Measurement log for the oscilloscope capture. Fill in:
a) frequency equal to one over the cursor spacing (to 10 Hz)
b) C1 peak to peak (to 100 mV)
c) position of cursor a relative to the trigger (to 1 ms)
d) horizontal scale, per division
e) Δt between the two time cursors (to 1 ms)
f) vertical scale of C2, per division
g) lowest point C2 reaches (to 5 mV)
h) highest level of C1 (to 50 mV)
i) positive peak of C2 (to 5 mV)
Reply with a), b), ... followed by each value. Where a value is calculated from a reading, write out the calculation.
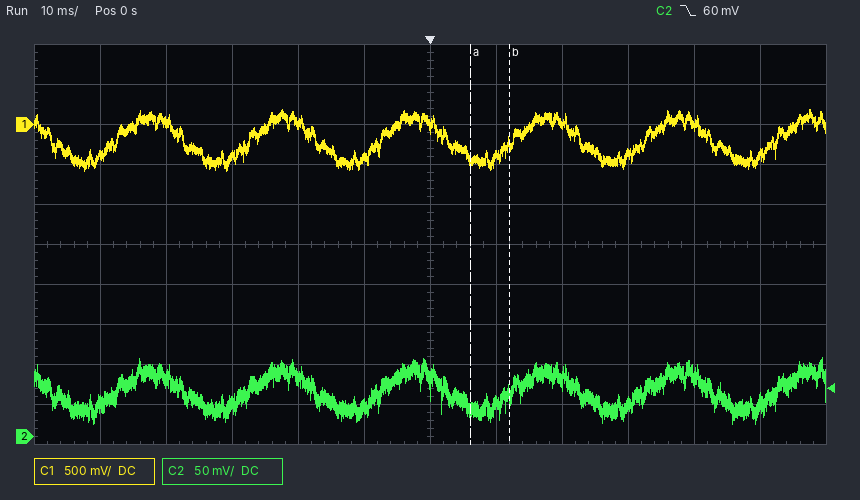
a) 1 / 6 ms ≈ 170 Hz
b) 800 mV
c) +6 ms
d) 10 ms
e) 6 ms
f) 50 mV
g) 15 mV
h) 200 mV
i) 100 mV
